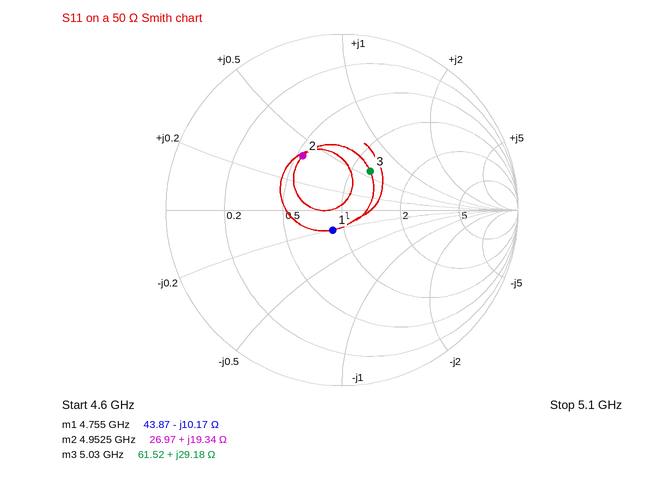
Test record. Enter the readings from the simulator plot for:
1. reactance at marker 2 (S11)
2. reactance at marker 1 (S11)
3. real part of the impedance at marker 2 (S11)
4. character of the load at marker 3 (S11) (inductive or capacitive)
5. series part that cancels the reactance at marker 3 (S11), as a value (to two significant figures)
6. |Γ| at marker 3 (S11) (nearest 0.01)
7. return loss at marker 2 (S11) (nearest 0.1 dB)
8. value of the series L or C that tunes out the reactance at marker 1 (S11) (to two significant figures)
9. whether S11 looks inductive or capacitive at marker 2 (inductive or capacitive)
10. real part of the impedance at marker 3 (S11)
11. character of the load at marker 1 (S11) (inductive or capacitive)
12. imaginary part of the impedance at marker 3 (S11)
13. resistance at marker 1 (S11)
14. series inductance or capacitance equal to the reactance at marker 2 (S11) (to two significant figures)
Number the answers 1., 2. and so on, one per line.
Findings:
1. +19.34 Ω
2. -10.17 Ω
3. 26.97 Ω
4. inductive
5. 1.1 pF
6. 0.27
7. 8.4 dB
8. 340 pH
9. inductive
10. 61.52 Ω
11. capacitive
12. +29.18 Ω
13. 43.87 Ω
14. 620 pH
